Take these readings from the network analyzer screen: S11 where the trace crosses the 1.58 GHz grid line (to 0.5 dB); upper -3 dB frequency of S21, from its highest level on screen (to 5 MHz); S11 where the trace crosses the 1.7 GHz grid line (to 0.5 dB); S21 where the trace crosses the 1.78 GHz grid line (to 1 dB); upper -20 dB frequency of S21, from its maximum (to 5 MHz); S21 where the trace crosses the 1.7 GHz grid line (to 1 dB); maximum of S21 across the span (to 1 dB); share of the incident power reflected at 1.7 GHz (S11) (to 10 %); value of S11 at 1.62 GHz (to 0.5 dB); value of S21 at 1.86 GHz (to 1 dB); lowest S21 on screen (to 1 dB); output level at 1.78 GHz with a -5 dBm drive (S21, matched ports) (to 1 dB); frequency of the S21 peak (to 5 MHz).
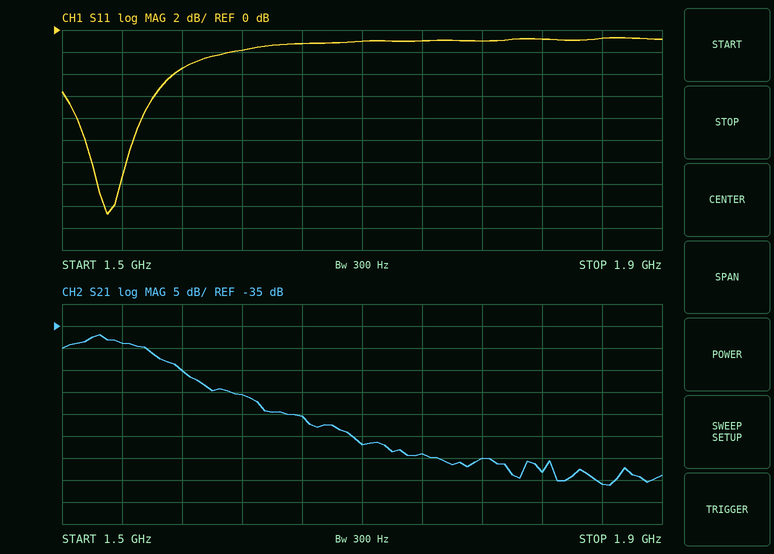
-3.5 dB
1.555 GHz
-1.0 dB
-65 dB
1.665 GHz
-62 dB
-37 dB
80 %
-2.0 dB
-71 dB
-71 dB
-70 dBm
1.525 GHz
